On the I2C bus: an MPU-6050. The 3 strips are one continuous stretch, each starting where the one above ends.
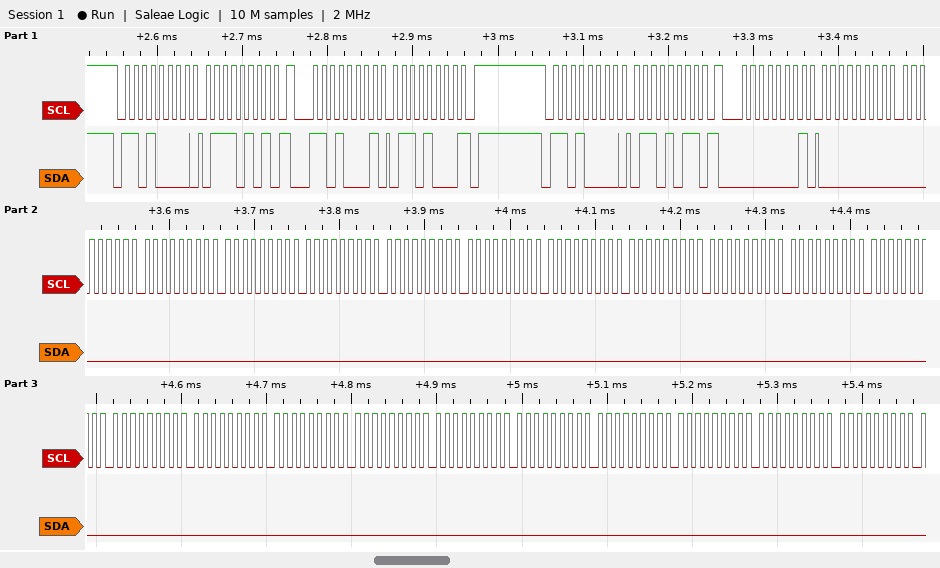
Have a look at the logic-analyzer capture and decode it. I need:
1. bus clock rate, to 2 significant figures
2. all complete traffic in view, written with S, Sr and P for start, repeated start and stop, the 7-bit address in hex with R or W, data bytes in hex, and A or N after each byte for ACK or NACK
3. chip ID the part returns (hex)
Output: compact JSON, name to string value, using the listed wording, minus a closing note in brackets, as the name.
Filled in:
{"bus clock rate, to 2 significant figures": "100 kHz", "all complete traffic in view, written with S, Sr and P for start, repeated start and stop, the 7-bit address in hex with R or W, data bytes in hex, and A or N after each byte for ACK or NACK": "S 68W A 75 A Sr 68R A 68 N P S 68W A 6B A Sr 00R A 00 A 00 A 00 A 00 A 00 A 00 A 00 A 00 A 00 A 00 A 00 A 00 A 00 A 00 A 00 A 00 A 00 A 00 A 00 A 00 A 00 A 00 A", "chip ID the part returns": "0x68"}
